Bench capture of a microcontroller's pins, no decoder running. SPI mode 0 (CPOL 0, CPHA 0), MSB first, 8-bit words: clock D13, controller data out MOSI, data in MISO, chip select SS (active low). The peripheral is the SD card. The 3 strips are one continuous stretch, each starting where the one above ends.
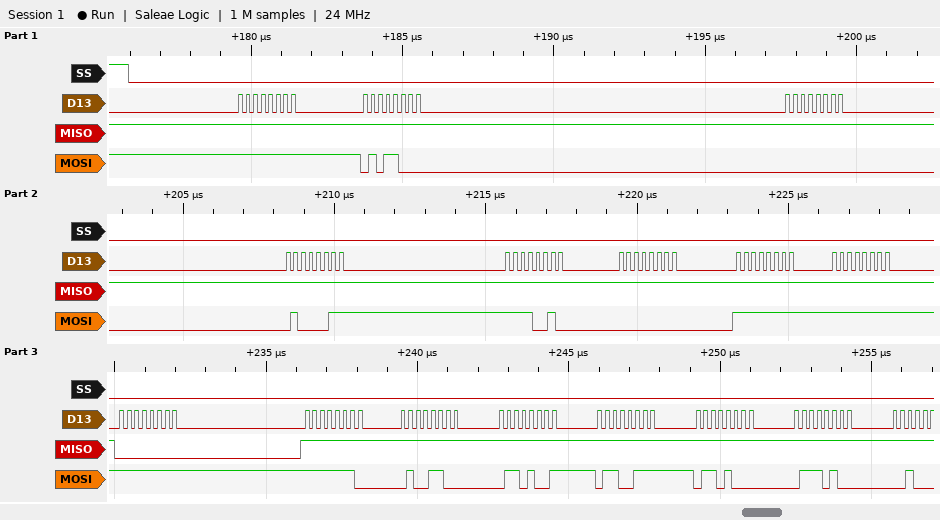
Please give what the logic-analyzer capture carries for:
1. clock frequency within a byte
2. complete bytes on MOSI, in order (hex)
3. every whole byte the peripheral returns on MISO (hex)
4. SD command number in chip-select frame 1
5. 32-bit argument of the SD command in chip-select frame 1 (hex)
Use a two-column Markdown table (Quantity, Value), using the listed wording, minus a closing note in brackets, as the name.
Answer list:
| Quantity | Value |
|---|---|
| clock frequency within a byte | 4 MHz |
| complete bytes on MOSI, in order | FF 58 00 43 F2 00 FF FF FF FE 4C 69 67 68 74 |
| every whole byte the peripheral returns on MISO | FF FF FF FF FF FF FF FF 00 FF FF FF FF FF FF |
| SD command number in chip-select frame 1 | CMD24 |
| 32-bit argument of the SD command in chip-select frame 1 | 0x0043F200 |
